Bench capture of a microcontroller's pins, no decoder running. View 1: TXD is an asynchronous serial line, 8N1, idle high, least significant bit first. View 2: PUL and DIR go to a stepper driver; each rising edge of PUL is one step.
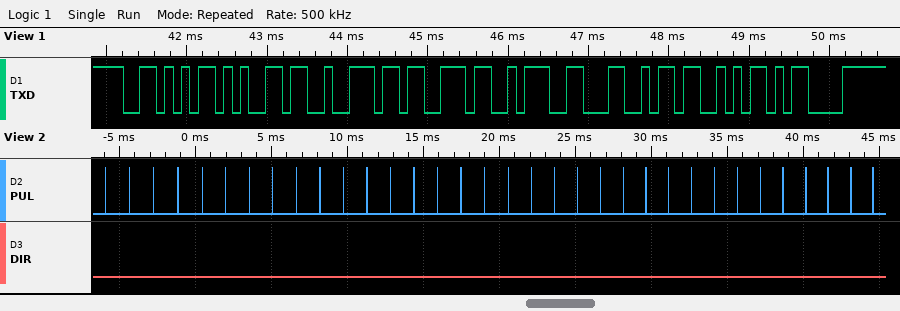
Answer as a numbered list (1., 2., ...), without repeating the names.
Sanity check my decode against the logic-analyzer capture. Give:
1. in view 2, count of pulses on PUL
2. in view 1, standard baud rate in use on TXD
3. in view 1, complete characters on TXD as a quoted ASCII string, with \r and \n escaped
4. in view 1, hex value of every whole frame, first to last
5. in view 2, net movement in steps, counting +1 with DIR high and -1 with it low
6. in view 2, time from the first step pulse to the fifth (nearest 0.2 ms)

1. 34
2. 9600 baud
3. "Vers:LS\r"
4. 56 65 72 73 3A 4C 53 0D
5. -34
6. 6.4 ms
